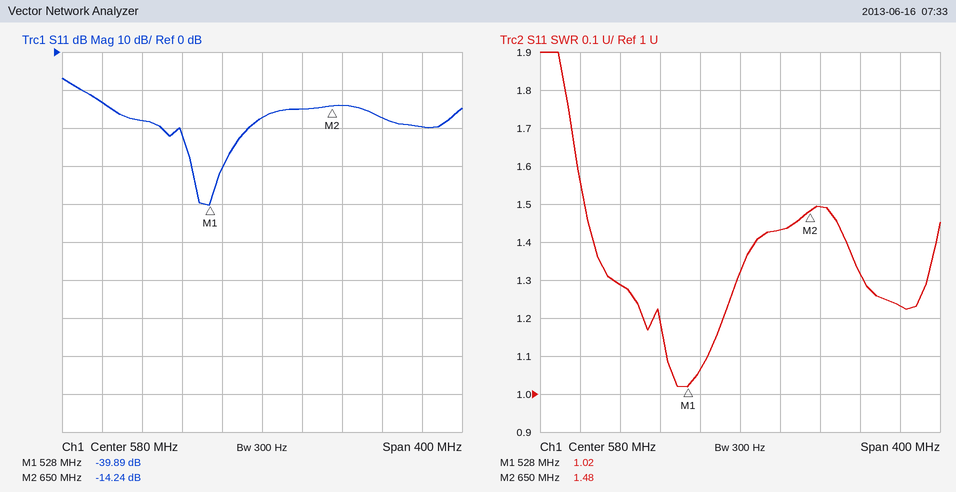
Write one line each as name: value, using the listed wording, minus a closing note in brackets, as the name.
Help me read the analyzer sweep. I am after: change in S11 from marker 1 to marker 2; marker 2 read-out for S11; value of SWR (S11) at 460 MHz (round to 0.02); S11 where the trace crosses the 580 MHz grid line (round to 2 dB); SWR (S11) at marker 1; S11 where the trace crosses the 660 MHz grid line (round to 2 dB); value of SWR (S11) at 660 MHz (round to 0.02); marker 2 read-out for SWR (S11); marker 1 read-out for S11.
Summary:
change in S11 from marker 1 to marker 2: 25.65 dB
marker 2 read-out for S11: -14.24 dB
value of SWR (S11) at 460 MHz: 1.28
S11 where the trace crosses the 580 MHz grid line: -18 dB
SWR (S11) at marker 1: 1.02
S11 where the trace crosses the 660 MHz grid line: -14 dB
value of SWR (S11) at 660 MHz: 1.50
marker 2 read-out for SWR: 1.48
marker 1 read-out for S11: -39.89 dB
